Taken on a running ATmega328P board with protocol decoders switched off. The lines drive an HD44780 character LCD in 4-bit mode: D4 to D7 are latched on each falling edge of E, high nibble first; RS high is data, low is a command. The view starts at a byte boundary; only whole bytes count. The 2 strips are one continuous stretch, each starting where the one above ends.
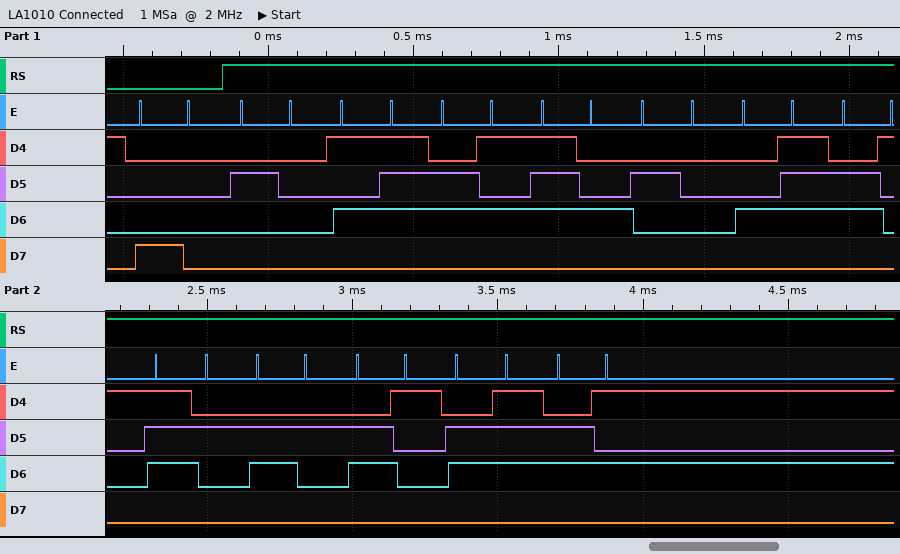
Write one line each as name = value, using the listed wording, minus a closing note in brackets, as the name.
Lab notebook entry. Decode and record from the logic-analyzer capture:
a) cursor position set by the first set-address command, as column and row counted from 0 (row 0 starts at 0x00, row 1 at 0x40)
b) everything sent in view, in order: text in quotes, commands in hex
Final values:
cursor position set by the first set-address command, as column and row counted from 0 = column 0, row 0
everything sent in view, in order: text in quotes, commands in hex = 0x80 " Wet Garbage"
